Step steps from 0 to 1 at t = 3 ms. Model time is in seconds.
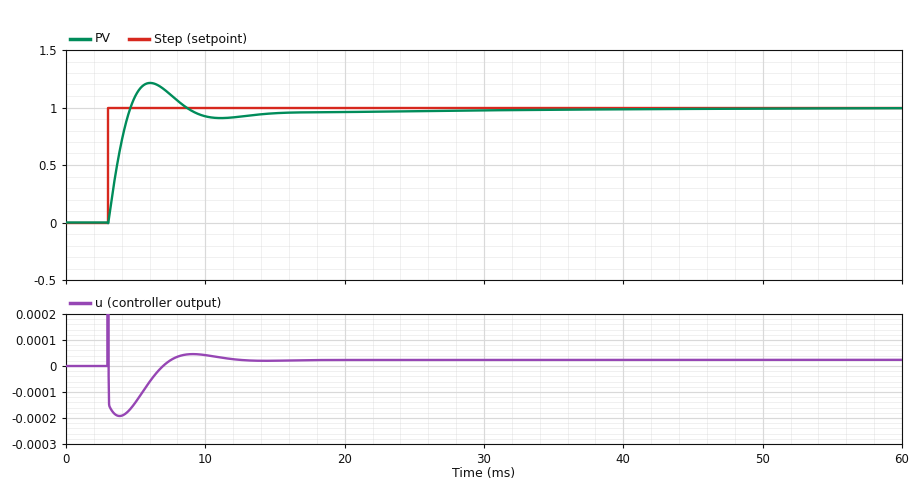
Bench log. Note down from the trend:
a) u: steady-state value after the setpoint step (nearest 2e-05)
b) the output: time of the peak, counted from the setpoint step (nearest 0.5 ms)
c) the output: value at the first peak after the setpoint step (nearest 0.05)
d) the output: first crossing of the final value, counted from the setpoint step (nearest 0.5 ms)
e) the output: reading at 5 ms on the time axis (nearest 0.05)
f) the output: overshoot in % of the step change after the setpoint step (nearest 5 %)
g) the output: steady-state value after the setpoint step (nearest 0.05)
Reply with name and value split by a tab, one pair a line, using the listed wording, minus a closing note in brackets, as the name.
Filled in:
u: steady-state value after the setpoint step	0.00002
the output: time of the peak, counted from the setpoint step	3.0 ms
the output: value at the first peak after the setpoint step	1.20
the output: first crossing of the final value, counted from the setpoint step	1.5 ms
the output: reading at 5 ms on the time axis	1.10
the output: overshoot in % of the step change after the setpoint step	20 %
the output: steady-state value after the setpoint step	1.00
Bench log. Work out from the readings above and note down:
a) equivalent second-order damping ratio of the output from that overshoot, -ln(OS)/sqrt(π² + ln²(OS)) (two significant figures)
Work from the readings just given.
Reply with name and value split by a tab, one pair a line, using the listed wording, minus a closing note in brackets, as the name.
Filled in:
equivalent second-order damping ratio of the output from that overshoot, -ln(OS)/sqrt(π² + ln²(OS))	0.46
